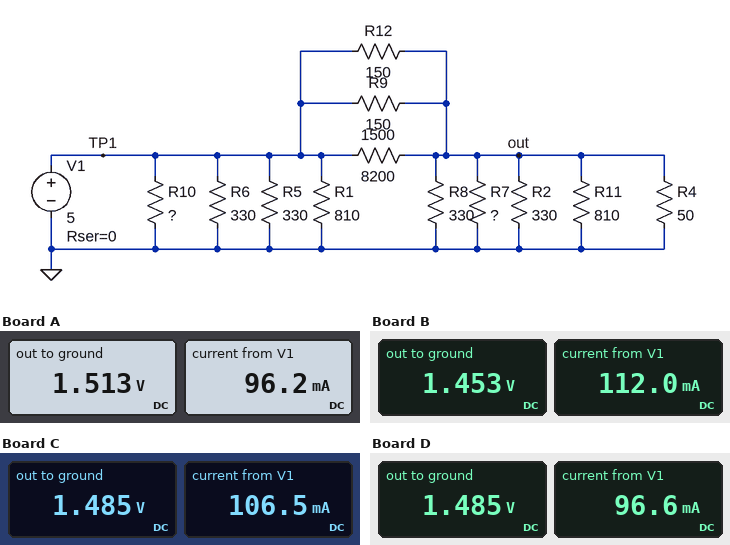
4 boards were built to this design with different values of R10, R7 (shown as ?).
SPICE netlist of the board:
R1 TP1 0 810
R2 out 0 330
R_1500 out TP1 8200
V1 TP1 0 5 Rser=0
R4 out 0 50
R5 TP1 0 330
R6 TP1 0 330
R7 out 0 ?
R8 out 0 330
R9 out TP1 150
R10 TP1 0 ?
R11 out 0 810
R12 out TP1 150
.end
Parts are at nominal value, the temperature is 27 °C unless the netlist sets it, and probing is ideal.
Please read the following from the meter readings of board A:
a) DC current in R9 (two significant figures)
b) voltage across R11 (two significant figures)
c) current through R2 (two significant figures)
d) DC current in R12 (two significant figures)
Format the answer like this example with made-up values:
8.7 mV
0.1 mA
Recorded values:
23 mA
1.5 V
4.6 mA
23 mA
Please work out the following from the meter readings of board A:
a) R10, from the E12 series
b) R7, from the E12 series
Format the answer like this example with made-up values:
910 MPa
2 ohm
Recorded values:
390 Ω
270 Ω
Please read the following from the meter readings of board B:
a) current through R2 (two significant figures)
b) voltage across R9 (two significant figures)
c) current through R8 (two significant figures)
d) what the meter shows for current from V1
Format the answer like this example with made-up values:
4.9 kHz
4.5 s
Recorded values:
4.4 mA
3.5 V
4.4 mA
112.0 mA
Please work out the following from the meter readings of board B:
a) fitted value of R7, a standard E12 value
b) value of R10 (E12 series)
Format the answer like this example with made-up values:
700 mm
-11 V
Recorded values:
180 Ω
180 Ω
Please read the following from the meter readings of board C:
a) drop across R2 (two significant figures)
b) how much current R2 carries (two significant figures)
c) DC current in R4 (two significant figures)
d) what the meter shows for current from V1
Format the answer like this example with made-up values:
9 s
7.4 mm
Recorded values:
1.5 V
4.5 mA
30 mA
106.5 mA
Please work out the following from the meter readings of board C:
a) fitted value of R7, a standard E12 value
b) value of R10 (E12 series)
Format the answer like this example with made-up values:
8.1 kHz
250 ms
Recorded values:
220 Ω
220 Ω
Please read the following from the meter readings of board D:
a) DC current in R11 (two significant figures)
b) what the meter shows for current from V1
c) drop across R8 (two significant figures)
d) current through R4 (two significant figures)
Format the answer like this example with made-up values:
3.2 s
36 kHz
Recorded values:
1.8 mA
96.6 mA
1.5 V
30 mA
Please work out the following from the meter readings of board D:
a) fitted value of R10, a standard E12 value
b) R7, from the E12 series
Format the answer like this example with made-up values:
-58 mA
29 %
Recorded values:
390 Ω
220 Ω
